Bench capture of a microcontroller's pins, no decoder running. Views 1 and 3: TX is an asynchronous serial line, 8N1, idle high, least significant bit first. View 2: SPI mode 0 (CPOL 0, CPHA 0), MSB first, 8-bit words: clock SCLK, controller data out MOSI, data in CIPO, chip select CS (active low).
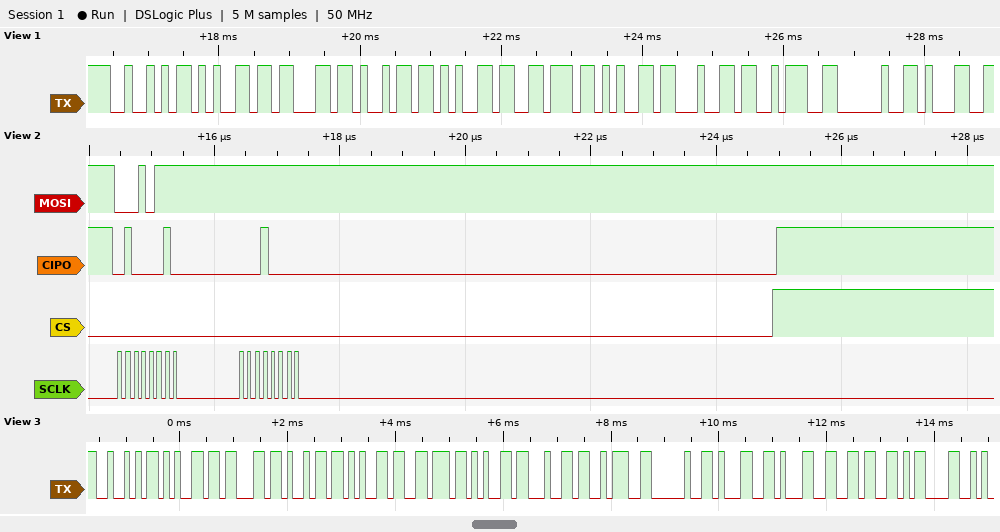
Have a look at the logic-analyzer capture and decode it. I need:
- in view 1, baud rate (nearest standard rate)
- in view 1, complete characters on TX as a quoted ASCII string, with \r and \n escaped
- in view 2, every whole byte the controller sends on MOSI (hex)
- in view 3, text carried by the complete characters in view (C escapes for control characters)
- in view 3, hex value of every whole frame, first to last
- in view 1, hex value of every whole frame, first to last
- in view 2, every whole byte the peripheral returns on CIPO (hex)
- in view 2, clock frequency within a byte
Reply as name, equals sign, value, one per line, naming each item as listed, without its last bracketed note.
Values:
in view 1, baud rate = 9600 baud
in view 1, complete characters on TX as a quoted ASCII string, with \r and \n escaped = "Recieved: 1"
in view 2, every whole byte the controller sends on MOSI = 0x17 0xFF
in view 3, text carried by the complete characters in view = "Recieved: 116\r"
in view 3, hex value of every whole frame, first to last = 52 65 63 69 65 76 65 64 3A 20 31 31 36 0D
in view 1, hex value of every whole frame, first to last = 52 65 63 69 65 76 65 64 3A 20 31
in view 2, every whole byte the peripheral returns on CIPO = 0x42 0x10
in view 2, clock frequency within a byte = 8 MHz
